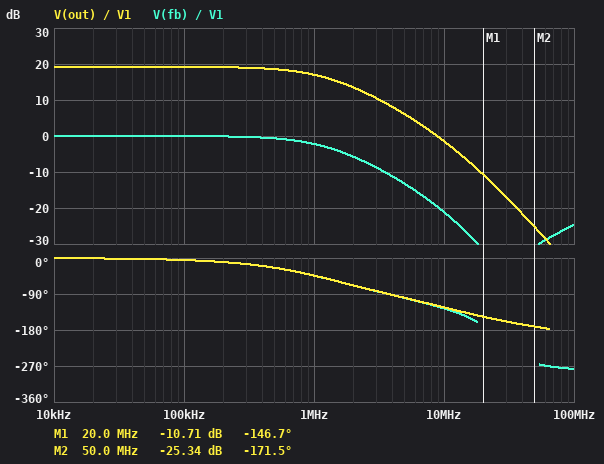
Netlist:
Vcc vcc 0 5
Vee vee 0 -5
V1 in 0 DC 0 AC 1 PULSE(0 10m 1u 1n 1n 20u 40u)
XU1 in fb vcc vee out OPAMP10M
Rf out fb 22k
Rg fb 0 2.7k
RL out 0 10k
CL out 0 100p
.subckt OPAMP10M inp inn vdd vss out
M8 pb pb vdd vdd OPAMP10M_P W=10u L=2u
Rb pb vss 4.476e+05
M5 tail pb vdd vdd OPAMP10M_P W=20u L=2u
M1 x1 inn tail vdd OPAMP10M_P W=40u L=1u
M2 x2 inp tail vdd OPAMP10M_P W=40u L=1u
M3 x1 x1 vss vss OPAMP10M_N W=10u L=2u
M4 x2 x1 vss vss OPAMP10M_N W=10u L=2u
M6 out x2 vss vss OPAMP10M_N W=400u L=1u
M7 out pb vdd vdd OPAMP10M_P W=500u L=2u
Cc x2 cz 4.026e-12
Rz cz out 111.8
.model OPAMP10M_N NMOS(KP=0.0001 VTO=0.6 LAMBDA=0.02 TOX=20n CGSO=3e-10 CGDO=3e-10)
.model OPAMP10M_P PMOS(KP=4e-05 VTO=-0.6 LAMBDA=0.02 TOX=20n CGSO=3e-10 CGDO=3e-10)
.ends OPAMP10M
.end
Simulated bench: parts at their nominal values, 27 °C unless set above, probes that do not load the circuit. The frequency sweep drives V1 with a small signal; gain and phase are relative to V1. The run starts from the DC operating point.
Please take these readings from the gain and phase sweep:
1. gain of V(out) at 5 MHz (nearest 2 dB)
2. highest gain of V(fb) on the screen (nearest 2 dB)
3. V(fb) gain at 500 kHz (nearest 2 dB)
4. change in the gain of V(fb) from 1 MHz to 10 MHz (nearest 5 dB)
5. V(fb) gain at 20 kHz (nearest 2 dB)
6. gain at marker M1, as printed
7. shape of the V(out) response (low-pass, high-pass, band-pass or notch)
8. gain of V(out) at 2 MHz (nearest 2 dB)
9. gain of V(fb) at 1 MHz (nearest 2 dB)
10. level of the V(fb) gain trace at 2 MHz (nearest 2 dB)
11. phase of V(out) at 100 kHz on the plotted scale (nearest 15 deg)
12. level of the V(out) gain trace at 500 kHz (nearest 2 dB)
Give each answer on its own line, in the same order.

6 dB
0 dB
0 dB
-20 dB
0 dB
-10.71 dB
low-pass
14 dB
-2 dB
-6 dB
0 deg
18 dB
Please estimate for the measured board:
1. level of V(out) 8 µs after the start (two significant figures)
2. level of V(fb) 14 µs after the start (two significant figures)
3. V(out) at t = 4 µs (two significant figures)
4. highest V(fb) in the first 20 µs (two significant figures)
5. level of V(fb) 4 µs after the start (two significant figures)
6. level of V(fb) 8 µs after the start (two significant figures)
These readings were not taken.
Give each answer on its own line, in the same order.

90 mV
9.8 mV
90 mV
9.8 mV
9.8 mV
9.8 mV
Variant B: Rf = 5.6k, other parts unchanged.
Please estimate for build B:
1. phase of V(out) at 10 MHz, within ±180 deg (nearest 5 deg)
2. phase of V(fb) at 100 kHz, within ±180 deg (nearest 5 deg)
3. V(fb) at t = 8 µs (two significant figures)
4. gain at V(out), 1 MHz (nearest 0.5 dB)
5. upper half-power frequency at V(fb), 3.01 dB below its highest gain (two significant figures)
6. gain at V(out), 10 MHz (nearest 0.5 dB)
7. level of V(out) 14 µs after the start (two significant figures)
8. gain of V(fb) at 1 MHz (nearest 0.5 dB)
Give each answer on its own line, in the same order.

-115 deg
0 deg
9.8 mV
9.5 dB
4.2 MHz
-0.5 dB
30 mV
0 dB
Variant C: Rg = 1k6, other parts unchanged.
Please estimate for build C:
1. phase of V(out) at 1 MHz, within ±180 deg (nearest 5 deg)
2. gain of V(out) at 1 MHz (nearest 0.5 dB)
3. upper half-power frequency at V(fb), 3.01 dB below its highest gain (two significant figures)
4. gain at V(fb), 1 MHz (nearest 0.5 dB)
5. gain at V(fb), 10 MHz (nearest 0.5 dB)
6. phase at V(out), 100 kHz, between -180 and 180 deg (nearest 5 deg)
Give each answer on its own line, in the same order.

-60 deg
19.0 dB
730 kHz
-4.5 dB
-25.5 dB
-10 deg
